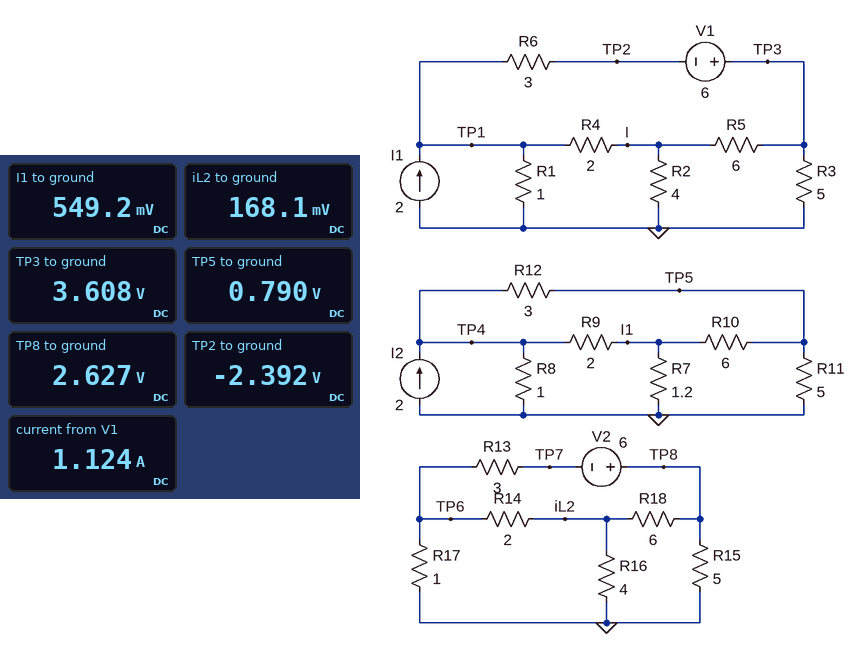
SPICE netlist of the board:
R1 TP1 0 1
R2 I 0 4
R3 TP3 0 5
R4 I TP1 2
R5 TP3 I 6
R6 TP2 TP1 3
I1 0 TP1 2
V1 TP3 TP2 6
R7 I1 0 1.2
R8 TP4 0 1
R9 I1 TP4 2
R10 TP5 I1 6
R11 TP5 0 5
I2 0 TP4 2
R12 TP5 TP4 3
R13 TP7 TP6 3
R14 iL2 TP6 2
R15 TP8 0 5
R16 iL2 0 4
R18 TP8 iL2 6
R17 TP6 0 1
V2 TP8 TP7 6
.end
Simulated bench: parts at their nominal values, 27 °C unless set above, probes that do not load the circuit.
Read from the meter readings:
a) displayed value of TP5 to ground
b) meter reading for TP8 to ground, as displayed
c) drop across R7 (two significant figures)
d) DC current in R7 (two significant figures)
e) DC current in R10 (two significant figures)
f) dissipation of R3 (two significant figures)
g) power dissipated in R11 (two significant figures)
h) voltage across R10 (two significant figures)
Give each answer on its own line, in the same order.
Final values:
0.790 V
2.627 V
550 mV
460 mA
40 mA
2.6 W
120 mW
240 mV
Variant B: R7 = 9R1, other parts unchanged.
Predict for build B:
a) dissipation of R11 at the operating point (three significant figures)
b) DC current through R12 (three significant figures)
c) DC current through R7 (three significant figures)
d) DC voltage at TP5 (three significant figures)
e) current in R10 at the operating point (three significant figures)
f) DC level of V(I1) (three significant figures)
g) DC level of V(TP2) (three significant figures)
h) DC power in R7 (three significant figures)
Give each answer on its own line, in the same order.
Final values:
237 mW
184 mA
142 mA
1.09 V
33.6 mA
1.29 V
-2.39 V
183 mW
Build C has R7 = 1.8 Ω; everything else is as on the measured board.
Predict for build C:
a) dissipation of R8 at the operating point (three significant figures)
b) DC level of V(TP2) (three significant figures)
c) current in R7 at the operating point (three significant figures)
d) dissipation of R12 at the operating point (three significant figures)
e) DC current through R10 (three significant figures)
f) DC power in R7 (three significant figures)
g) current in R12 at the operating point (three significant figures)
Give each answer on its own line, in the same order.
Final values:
2.07 W
-2.39 V
391 mA
114 mW
24.7 mA
276 mW
195 mA
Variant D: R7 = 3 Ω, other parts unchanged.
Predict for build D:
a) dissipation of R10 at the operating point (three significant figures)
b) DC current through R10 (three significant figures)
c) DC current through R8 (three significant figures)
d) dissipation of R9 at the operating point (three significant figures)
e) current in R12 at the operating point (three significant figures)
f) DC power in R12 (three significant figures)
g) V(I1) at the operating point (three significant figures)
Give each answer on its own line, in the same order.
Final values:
104 µW
4.16 mA
1.51 A
179 mW
191 mA
110 mW
911 mV
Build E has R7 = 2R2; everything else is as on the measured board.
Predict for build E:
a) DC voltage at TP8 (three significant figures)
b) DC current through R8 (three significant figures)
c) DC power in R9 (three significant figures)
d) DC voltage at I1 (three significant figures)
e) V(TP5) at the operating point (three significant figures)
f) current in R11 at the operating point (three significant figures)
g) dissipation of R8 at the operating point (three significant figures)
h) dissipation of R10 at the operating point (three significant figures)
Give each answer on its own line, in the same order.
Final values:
2.63 V
1.47 A
232 mW
785 mV
885 mV
177 mA
2.15 W
1.66 mW
